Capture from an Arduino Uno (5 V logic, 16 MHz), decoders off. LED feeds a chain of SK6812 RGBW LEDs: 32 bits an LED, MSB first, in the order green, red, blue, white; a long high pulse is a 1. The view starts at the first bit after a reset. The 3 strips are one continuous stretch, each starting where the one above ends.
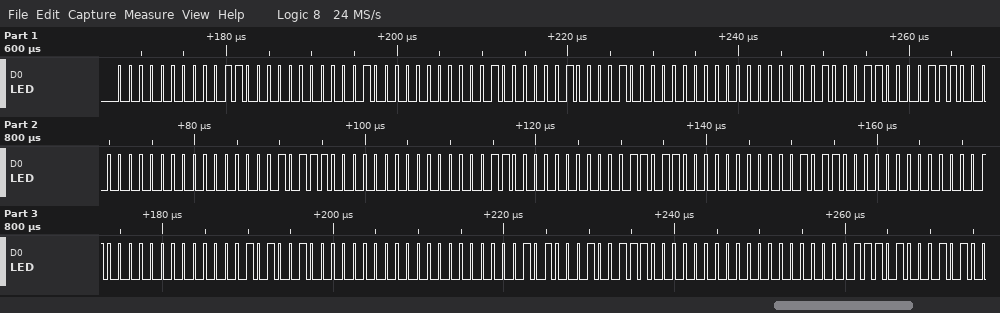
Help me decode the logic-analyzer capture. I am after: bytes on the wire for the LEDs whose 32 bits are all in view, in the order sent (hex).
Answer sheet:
00 30 01 00 10 21 00 00 23 0E 00 00 2E 00 03 00 1B 00 16 00 08 00 29 00 00 0A 27 00
